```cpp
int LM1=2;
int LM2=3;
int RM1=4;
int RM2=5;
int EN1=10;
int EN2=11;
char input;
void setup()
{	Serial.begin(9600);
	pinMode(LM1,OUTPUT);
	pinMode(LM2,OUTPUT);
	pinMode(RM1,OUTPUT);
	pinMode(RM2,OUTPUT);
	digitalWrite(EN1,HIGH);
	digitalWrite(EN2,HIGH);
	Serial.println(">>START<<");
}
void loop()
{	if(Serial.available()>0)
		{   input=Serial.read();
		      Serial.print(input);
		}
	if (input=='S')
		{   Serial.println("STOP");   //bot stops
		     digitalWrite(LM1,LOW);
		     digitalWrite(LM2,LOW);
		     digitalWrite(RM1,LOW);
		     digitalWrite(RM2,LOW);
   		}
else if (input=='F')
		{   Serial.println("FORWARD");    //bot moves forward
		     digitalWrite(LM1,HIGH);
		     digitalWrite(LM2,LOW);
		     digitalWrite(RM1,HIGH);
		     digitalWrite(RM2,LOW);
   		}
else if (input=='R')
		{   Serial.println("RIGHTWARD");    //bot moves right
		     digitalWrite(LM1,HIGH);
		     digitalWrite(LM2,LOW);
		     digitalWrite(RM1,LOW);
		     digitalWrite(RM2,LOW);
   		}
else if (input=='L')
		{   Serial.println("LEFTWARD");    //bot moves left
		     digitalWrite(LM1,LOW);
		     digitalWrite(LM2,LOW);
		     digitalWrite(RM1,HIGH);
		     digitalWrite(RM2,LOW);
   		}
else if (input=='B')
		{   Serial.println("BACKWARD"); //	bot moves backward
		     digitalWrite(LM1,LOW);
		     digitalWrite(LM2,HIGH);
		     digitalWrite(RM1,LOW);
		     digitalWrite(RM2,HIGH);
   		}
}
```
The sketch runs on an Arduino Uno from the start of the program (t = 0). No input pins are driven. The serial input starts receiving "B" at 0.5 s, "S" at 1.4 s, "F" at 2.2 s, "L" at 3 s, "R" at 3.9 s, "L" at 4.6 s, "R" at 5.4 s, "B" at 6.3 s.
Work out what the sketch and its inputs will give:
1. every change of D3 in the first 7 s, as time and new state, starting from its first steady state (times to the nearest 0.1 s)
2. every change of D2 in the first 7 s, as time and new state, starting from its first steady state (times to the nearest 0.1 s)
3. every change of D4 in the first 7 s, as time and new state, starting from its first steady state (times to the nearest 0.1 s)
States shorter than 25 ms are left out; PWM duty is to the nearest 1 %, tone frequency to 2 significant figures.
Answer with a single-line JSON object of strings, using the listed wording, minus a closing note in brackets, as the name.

{"every change of D3 in the first 7 s, as time and new state, starting from its first steady state": "0 s low; 0.5 s high; 1.4 s low; 6.3 s high", "every change of D2 in the first 7 s, as time and new state, starting from its first steady state": "0 s low; 2.2 s high; 3 s low; 3.9 s high; 4.6 s low; 5.4 s high; 6.3 s low", "every change of D4 in the first 7 s, as time and new state, starting from its first steady state": "0 s low; 2.2 s high; 3.9 s low; 4.6 s high; 5.4 s low"}
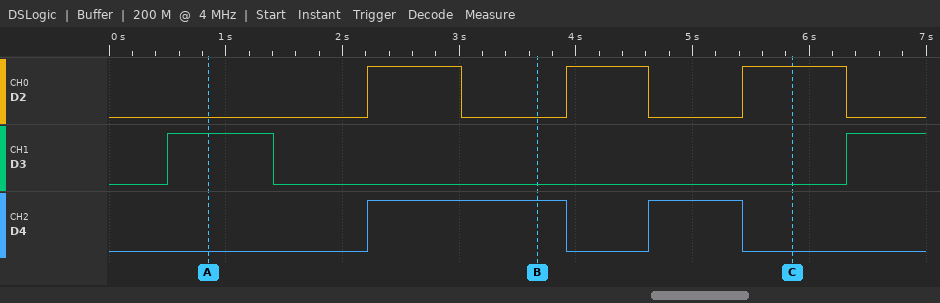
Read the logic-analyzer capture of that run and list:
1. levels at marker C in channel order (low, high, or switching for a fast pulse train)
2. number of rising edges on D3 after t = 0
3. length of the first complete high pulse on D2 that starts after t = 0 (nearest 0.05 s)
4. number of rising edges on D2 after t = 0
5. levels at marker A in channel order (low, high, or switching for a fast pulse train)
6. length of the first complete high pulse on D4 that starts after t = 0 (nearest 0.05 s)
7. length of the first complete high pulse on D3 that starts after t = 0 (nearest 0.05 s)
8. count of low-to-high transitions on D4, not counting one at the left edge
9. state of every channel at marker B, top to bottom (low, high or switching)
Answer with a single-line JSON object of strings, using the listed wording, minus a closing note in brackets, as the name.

{"levels at marker C in channel order": "D2 high, D3 low, D4 low", "number of rising edges on D3 after t = 0": "2", "length of the first complete high pulse on D2 that starts after t = 0": "0.80 s", "number of rising edges on D2 after t = 0": "3", "levels at marker A in channel order": "D2 low, D3 high, D4 low", "length of the first complete high pulse on D4 that starts after t = 0": "1.70 s", "length of the first complete high pulse on D3 that starts after t = 0": "0.90 s", "count of low-to-high transitions on D4, not counting one at the left edge": "2", "state of every channel at marker B, top to bottom": "D2 low, D3 low, D4 high"}
